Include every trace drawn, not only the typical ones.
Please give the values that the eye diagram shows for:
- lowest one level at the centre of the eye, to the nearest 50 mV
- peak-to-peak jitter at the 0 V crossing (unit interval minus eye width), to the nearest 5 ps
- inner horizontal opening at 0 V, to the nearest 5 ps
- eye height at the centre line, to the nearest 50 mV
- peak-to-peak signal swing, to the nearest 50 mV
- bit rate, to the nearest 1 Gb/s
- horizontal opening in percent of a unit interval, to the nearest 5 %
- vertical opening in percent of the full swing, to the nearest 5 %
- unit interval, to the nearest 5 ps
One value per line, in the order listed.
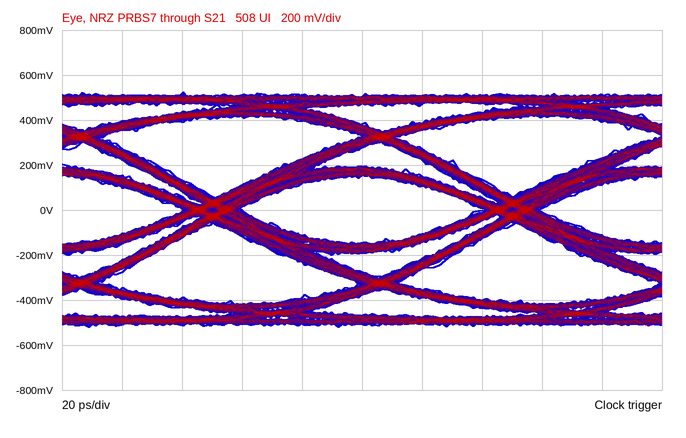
150 mV
20 ps
80 ps
300 mV
1.05 V
10 Gb/s
80 %
30 %
100 ps
